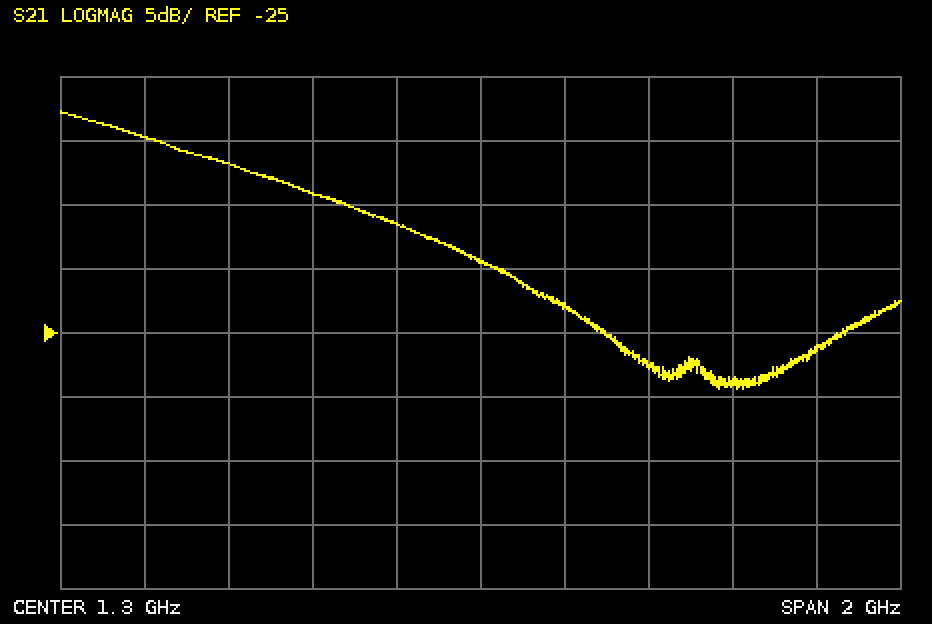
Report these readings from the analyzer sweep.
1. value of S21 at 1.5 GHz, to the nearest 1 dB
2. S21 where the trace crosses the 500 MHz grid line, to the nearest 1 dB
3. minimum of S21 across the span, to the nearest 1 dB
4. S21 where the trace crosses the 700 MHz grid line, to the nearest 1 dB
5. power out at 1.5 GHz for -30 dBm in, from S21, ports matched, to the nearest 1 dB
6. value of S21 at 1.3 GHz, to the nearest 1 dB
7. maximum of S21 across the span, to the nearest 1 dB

-23 dB
-10 dB
-29 dB
-12 dB
-53 dBm
-19 dB
-8 dB
